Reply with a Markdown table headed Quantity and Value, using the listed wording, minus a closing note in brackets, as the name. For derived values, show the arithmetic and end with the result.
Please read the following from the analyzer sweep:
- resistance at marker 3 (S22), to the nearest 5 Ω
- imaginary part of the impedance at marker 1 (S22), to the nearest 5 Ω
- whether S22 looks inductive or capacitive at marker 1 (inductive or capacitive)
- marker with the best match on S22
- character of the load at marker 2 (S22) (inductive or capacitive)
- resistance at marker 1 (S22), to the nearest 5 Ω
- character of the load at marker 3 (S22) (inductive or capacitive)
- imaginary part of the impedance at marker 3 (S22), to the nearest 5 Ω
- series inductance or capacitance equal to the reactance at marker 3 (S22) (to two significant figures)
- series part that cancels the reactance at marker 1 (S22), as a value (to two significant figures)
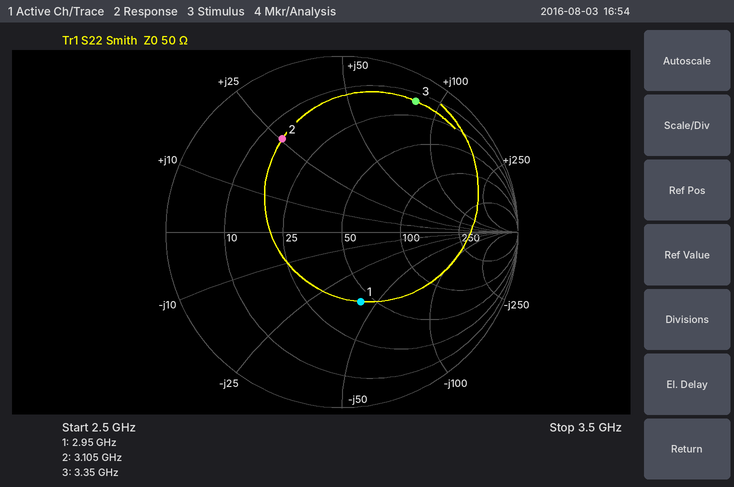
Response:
| Quantity | Value |
|---|---|
| resistance at marker 3 (S22), to the nearest 5 Ω | 15 Ω |
| imaginary part of the impedance at marker 1 (S22), to the nearest 5 Ω | -40 Ω |
| whether S22 looks inductive or capacitive at marker 1 | capacitive |
| marker with the best match on S22 | marker 1 |
| character of the load at marker 2 (S22) | inductive |
| resistance at marker 1 (S22), to the nearest 5 Ω | 45 Ω |
| character of the load at marker 3 (S22) | inductive |
| imaginary part of the impedance at marker 3 (S22), to the nearest 5 Ω | +85 Ω |
| series inductance or capacitance equal to the reactance at marker 3 (S22) | L = 85 Ω/(2π × 3.35 GHz) ≈ 4.0 nH |
| series part that cancels the reactance at marker 1 (S22), as a value | L = 40 Ω/(2π × 2.95 GHz) ≈ 2.2 nH |
